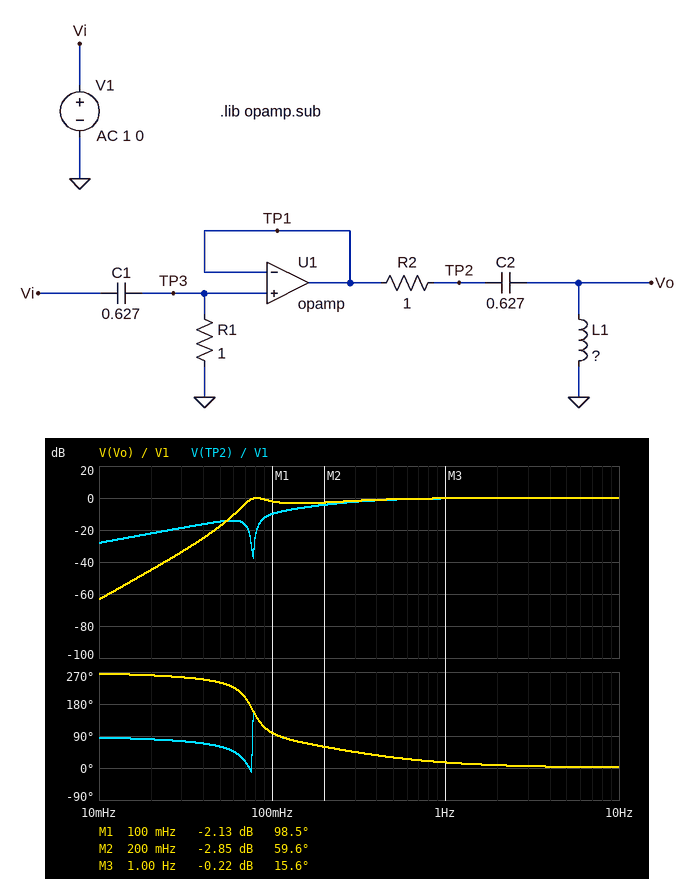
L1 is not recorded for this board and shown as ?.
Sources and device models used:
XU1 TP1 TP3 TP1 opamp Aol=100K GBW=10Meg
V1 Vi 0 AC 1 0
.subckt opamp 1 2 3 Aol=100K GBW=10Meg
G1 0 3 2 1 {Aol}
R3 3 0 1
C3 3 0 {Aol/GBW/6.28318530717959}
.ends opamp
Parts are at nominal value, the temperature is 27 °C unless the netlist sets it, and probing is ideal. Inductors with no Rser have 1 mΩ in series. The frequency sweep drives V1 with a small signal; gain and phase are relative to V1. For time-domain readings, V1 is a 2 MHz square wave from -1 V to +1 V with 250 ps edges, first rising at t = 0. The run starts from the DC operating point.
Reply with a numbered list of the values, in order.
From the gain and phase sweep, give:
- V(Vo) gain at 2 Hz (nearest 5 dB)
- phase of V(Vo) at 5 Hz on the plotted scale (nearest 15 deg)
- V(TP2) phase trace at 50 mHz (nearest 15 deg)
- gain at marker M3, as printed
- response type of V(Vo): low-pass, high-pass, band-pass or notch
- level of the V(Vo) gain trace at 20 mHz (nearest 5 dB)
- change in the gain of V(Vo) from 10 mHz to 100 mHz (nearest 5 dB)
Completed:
1. 0 dB
2. 0 deg
3. 60 deg
4. -0.22 dB
5. high-pass
6. -45 dB
7. 60 dB
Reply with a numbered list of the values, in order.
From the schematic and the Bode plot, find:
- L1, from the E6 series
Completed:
1. 6.8 H
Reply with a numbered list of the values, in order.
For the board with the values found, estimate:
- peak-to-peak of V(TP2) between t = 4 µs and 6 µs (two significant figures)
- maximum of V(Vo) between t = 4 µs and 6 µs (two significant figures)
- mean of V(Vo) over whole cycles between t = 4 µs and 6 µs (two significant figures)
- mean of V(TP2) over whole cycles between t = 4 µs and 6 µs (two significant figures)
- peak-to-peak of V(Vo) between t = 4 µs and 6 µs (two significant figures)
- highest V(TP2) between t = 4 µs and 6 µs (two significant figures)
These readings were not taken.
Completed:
1. 2.0 V
2. 2.0 V
3. 1.0 V
4. 1.0 V
5. 2.0 V
6. 2.0 V
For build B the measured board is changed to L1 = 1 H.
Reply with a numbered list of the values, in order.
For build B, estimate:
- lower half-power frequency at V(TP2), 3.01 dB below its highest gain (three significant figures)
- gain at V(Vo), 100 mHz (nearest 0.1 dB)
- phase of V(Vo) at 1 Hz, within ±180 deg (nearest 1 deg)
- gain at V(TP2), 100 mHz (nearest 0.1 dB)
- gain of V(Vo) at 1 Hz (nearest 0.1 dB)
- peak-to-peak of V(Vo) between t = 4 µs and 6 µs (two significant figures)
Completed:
1. 372 mHz
2. -19.4 dB
3. 24 deg
4. -9.8 dB
5. 0 dB
6. 2.0 V
